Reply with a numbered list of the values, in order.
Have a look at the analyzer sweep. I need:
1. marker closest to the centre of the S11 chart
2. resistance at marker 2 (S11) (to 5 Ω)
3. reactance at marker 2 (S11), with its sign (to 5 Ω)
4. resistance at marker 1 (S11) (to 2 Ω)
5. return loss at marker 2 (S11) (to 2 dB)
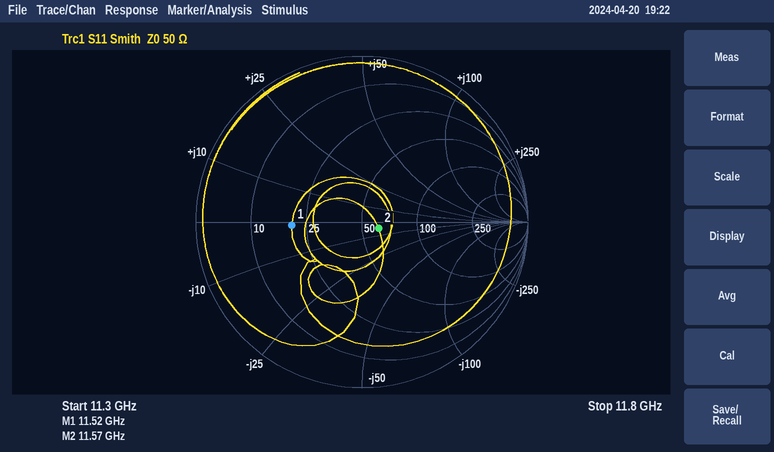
1. marker 2
2. 60 Ω
3. -5 Ω
4. 20 Ω
5. 20 dB
